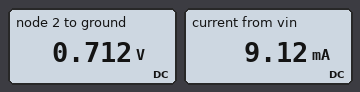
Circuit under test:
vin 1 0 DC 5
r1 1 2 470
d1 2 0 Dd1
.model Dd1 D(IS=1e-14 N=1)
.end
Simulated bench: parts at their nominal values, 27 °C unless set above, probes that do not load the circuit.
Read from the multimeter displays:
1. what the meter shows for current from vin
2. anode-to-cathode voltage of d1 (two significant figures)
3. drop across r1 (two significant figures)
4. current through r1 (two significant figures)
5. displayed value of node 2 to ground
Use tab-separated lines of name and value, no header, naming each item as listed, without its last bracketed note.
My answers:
what the meter shows for current from vin	9.12 mA
anode-to-cathode voltage of d1	710 mV
drop across r1	4.3 V
current through r1	9.1 mA
displayed value of node 2 to ground	0.712 V
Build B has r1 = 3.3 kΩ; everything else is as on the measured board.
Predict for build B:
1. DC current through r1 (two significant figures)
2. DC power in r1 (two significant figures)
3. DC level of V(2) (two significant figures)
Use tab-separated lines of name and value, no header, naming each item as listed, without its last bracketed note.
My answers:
DC current through r1	1.3 mA
DC power in r1	5.7 mW
DC level of V(2)	660 mV
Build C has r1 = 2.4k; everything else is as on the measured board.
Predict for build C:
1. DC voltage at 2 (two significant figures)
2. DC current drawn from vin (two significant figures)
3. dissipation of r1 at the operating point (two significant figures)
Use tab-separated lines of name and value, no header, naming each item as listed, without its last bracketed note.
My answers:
DC voltage at 2	670 mV
DC current drawn from vin	1.8 mA
dissipation of r1 at the operating point	7.8 mW
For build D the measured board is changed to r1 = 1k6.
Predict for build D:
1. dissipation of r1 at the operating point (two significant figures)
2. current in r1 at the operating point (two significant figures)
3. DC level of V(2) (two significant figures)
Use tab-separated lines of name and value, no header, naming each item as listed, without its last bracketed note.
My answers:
dissipation of r1 at the operating point	12 mW
current in r1 at the operating point	2.7 mA
DC level of V(2)	680 mV
